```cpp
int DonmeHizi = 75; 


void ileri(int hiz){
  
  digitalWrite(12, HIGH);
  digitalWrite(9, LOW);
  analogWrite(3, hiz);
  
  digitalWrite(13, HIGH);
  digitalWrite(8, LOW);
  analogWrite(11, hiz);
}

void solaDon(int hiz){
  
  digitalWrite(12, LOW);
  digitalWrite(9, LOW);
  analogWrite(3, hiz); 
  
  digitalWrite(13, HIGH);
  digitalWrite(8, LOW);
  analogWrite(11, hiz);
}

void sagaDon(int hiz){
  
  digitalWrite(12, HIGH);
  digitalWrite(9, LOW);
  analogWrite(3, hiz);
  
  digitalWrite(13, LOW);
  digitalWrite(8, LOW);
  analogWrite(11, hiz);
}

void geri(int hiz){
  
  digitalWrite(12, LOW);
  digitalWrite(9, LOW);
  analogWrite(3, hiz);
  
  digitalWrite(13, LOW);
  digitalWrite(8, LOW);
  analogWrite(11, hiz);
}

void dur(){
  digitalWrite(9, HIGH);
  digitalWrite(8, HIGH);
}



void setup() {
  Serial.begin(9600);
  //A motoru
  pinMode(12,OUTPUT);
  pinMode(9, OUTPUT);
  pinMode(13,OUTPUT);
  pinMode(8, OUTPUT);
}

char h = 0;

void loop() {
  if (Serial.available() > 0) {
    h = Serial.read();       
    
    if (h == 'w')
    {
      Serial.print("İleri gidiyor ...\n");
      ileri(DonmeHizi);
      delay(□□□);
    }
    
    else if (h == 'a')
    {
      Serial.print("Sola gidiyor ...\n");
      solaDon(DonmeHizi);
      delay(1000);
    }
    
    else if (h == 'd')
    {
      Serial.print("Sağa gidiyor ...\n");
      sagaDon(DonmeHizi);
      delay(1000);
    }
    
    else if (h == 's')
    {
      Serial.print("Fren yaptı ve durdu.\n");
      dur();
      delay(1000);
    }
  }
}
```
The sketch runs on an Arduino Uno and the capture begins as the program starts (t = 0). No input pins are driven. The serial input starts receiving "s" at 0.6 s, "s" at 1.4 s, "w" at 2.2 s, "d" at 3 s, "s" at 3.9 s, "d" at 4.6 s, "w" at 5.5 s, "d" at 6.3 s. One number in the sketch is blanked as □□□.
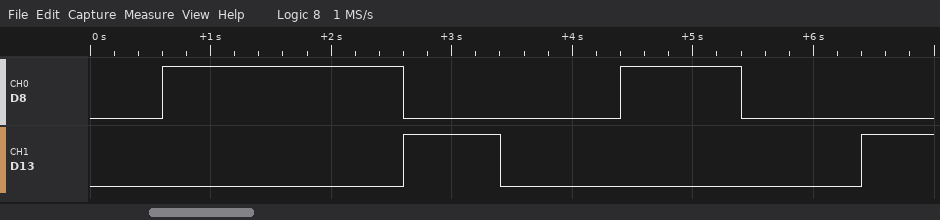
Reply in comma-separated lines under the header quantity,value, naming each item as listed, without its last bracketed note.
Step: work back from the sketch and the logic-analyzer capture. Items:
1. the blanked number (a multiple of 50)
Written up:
quantity,value
the blanked number,800
